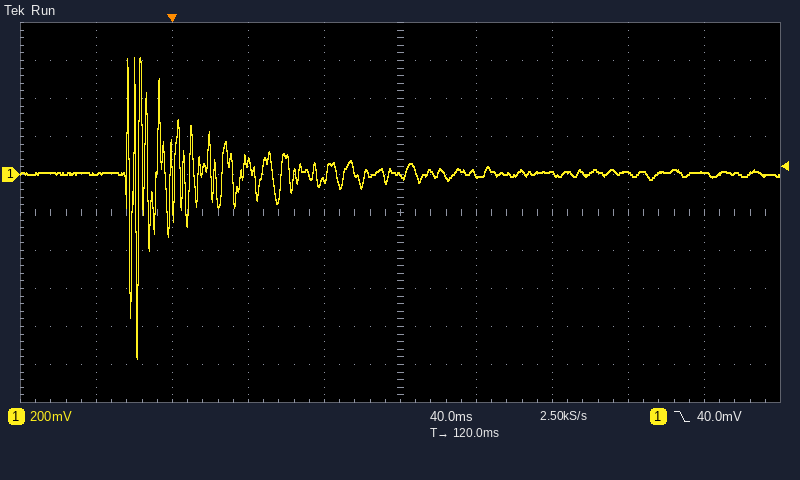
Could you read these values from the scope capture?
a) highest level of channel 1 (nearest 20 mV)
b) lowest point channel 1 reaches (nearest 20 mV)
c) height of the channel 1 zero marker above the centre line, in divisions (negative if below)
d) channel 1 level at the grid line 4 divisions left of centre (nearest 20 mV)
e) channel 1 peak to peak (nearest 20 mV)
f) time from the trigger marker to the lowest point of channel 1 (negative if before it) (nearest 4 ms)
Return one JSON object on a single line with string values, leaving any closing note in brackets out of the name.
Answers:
{"highest level of channel 1": "620 mV", "lowest point channel 1 reaches": "-960 mV", "height of the channel 1 zero marker above the centre line, in divisions": "+1.0 div", "channel 1 level at the grid line 4 divisions left of centre": "0 mV", "channel 1 peak to peak": "1.58 V", "time from the trigger marker to the lowest point of channel 1 (negative if before it)": "-20 ms"}
